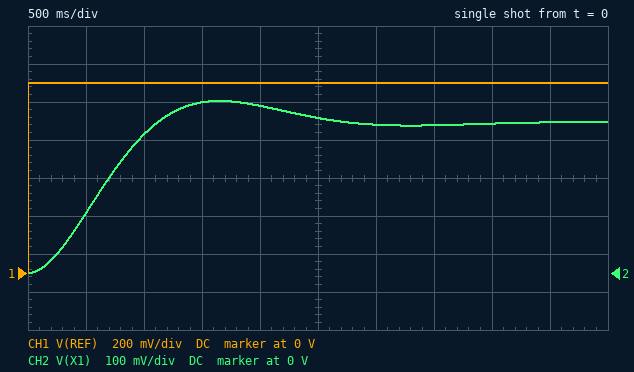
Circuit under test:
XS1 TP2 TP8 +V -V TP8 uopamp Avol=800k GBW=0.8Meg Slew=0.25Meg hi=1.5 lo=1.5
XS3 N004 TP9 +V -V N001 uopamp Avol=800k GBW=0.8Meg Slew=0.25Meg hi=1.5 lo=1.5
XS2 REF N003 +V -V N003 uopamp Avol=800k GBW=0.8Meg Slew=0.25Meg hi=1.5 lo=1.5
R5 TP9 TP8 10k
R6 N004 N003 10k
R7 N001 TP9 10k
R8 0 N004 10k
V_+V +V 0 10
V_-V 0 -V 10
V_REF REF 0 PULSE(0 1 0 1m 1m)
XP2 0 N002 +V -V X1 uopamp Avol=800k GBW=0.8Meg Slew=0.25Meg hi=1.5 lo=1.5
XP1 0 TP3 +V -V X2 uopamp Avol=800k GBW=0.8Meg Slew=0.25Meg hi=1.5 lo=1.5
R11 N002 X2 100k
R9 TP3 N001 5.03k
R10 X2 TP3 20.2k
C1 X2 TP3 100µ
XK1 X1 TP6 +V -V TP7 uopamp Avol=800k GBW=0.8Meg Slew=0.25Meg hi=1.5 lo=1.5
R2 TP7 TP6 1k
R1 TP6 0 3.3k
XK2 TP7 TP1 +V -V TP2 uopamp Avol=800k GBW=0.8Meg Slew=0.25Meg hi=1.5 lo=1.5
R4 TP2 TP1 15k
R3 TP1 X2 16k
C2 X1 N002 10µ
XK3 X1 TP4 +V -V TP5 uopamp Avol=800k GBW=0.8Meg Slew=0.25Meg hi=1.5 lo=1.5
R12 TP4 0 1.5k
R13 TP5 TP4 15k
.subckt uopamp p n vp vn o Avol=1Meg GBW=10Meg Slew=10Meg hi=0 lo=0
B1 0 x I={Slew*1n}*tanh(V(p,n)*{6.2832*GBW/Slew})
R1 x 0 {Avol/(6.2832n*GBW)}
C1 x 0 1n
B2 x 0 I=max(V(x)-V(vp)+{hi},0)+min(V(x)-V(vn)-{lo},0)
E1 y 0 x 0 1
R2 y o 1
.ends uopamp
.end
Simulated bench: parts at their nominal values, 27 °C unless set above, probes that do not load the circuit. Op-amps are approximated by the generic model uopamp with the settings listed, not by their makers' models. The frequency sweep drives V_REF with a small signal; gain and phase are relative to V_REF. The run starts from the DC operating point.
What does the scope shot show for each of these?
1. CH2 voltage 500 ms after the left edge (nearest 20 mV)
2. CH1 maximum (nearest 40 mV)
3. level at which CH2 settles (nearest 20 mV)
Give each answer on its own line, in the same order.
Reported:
160 mV
1.00 V
400 mV
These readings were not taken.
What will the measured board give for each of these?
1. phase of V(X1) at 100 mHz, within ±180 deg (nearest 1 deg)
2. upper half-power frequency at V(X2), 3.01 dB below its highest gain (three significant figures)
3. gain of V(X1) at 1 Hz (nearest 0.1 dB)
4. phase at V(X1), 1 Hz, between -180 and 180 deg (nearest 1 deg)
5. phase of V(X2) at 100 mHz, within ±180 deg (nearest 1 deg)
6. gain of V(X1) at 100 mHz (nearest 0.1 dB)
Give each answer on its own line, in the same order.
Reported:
-18 deg
591 mHz
-25.5 dB
-157 deg
-108 deg
-7.8 dB
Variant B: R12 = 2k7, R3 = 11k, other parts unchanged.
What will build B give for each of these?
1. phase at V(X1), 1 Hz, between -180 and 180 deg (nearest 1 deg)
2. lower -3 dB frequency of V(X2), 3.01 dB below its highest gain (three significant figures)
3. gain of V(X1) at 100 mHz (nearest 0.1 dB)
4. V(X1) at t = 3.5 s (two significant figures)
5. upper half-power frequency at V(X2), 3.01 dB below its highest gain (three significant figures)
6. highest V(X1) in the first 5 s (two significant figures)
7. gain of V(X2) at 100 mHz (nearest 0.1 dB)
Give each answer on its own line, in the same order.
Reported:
-149 deg
214 mHz
-9.7 dB
320 mV
724 mHz
350 mV
-13.7 dB
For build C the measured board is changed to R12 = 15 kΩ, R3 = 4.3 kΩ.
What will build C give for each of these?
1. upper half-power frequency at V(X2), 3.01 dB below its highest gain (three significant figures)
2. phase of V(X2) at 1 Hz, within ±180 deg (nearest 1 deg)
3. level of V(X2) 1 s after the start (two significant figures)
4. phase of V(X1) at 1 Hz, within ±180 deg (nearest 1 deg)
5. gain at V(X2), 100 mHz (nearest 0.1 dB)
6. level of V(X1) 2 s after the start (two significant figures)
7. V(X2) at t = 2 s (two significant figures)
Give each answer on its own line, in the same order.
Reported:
1.39 Hz
149 deg
-68 mV
-121 deg
-19.8 dB
170 mV
-7.6 mV
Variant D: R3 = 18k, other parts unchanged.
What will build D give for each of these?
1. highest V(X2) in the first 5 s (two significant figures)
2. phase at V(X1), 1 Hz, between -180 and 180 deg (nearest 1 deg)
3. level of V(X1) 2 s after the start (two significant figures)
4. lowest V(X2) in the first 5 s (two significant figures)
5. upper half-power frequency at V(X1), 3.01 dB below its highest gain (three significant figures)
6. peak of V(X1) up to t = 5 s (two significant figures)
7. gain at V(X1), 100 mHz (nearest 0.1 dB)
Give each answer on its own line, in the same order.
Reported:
84 mV
-159 deg
470 mV
-500 mV
406 mHz
490 mV
-7.2 dB
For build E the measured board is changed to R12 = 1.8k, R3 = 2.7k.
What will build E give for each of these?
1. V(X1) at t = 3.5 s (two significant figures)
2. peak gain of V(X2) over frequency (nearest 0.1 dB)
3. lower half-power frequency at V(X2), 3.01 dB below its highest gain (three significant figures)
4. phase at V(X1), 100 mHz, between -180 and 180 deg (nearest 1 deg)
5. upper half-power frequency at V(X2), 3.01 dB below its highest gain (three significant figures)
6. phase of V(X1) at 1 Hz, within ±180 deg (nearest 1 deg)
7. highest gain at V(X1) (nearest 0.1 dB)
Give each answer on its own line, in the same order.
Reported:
120 mV
-15.3 dB
210 mHz
-24 deg
2.05 Hz
-107 deg
-18.6 dB
